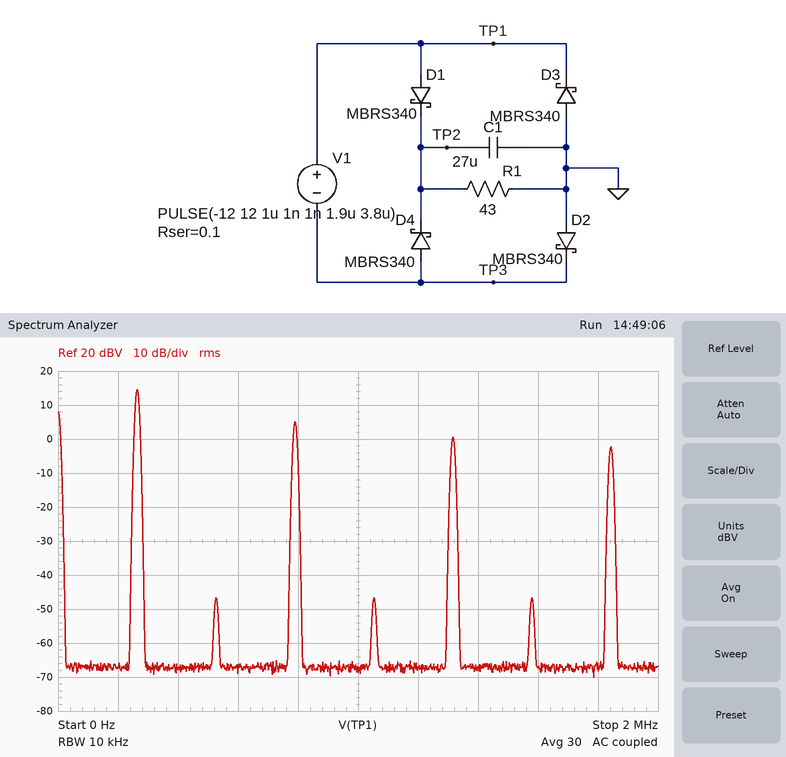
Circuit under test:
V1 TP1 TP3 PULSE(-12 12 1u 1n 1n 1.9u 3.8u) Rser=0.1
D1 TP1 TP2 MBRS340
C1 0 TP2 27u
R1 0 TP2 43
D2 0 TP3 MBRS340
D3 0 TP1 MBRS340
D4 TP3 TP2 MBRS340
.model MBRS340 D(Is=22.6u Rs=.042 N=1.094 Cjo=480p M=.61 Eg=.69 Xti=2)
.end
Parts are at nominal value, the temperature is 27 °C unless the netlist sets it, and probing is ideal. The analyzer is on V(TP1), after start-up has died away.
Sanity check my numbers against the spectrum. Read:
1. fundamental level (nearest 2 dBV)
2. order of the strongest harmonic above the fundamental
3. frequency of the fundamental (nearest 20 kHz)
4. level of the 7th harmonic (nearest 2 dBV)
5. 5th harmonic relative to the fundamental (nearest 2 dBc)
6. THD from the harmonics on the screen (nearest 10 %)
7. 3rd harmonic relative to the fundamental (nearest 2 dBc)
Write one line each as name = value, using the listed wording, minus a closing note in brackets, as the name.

fundamental level = 14 dBV
order of the strongest harmonic above the fundamental = 3
frequency of the fundamental = 260 kHz
level of the 7th harmonic = -2 dBV
5th harmonic relative to the fundamental = -14 dBc
THD from the harmonics on the screen = 40 %
3rd harmonic relative to the fundamental = -10 dBc
